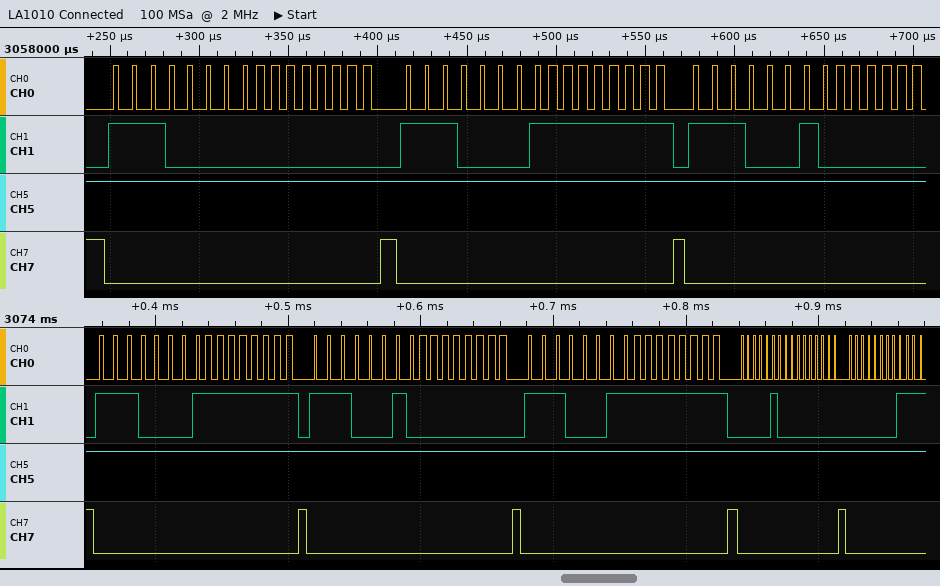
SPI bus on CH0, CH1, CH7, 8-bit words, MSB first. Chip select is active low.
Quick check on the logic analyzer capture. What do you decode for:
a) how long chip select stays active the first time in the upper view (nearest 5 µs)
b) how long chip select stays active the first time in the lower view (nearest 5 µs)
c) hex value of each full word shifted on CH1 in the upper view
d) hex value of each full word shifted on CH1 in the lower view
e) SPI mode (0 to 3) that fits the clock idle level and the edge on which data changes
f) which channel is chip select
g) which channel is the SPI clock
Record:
155 µs
155 µs
E0, 00, E1, FF, E2
E1, FF, E2, 00, E3, FF, 04, 00, 00
1
CH7
CH0
